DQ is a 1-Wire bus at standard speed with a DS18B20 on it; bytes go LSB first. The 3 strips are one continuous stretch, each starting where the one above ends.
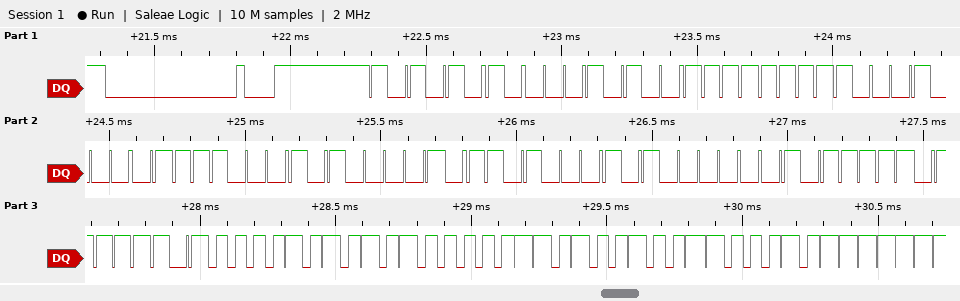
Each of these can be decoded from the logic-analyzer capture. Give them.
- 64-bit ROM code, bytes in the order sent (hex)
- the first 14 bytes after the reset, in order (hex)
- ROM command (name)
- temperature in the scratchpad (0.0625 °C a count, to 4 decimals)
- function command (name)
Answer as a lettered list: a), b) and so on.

a) 28 FF 11 1E 85 16 05 FA
b) 55 28 FF 11 1E 85 16 05 FA BE 50 05 4B 46
c) Match ROM
d) 85.0000 °C
e) Read Scratchpad
